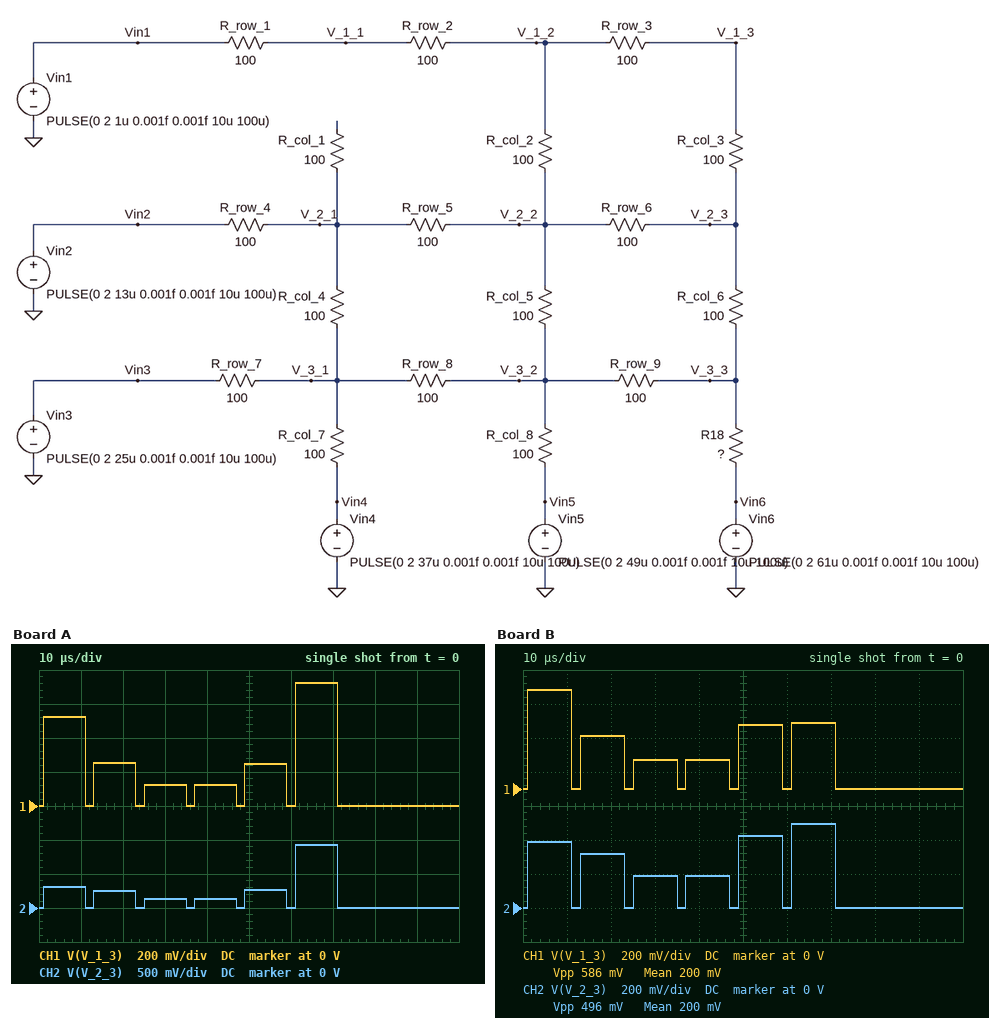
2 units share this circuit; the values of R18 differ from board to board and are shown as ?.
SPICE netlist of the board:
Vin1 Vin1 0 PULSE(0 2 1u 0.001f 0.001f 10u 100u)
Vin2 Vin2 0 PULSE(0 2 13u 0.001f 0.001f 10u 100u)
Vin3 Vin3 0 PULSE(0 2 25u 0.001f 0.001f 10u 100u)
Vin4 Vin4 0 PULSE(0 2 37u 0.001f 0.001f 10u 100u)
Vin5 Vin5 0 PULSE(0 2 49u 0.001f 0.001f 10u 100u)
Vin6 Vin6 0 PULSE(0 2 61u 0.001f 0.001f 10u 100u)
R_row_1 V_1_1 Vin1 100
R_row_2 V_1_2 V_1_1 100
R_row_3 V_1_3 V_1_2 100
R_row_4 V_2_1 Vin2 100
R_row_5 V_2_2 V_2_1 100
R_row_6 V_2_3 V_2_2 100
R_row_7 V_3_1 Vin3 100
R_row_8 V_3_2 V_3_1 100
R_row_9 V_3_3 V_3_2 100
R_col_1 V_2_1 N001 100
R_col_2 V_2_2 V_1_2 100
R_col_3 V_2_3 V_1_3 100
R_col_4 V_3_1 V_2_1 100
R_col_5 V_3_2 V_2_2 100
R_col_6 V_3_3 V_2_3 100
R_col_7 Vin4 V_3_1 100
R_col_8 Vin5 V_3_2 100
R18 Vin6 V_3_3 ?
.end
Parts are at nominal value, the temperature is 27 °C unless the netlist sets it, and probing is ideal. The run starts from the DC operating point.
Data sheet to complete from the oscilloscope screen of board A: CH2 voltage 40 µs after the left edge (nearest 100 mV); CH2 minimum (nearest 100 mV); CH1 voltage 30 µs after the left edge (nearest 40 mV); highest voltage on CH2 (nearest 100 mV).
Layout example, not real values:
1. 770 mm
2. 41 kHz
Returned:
1. 100 mV
2. 0 V
3. 120 mV
4. 900 mV
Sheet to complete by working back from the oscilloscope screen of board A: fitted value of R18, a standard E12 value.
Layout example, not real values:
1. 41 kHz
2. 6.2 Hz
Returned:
1. 33 Ω
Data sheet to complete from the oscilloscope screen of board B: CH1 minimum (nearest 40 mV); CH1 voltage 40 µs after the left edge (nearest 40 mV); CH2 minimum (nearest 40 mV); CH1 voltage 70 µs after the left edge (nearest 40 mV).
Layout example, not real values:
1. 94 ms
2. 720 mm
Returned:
1. 0 V
2. 160 mV
3. 0 V
4. 400 mV
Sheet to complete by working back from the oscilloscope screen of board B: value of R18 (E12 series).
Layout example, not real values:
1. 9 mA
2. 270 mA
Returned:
1. 150 Ω
